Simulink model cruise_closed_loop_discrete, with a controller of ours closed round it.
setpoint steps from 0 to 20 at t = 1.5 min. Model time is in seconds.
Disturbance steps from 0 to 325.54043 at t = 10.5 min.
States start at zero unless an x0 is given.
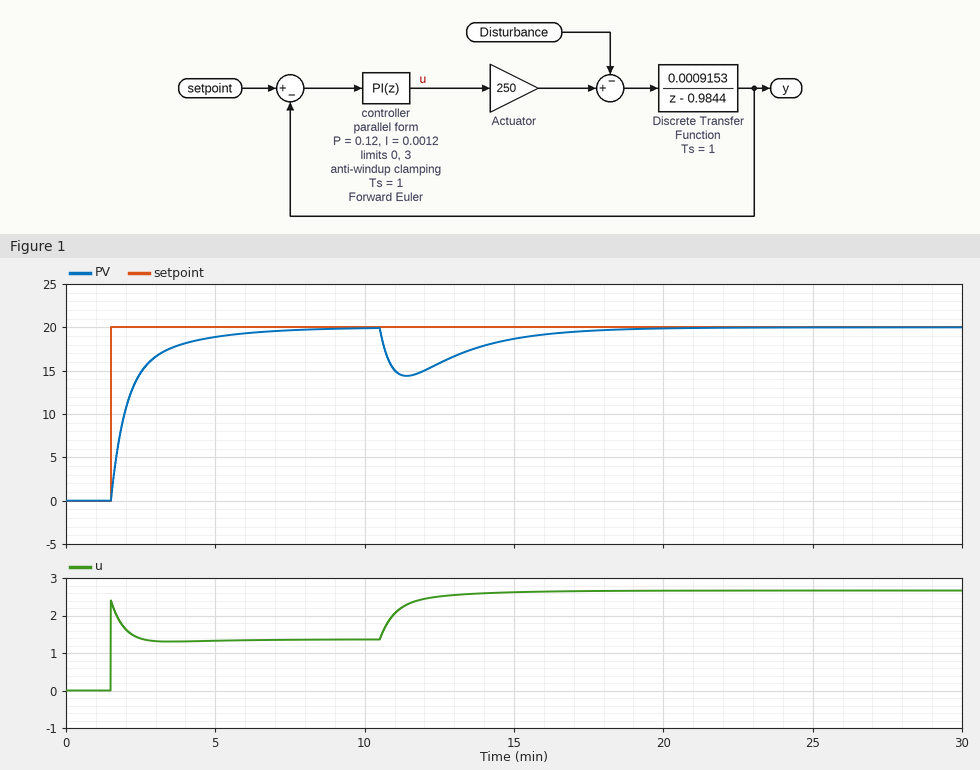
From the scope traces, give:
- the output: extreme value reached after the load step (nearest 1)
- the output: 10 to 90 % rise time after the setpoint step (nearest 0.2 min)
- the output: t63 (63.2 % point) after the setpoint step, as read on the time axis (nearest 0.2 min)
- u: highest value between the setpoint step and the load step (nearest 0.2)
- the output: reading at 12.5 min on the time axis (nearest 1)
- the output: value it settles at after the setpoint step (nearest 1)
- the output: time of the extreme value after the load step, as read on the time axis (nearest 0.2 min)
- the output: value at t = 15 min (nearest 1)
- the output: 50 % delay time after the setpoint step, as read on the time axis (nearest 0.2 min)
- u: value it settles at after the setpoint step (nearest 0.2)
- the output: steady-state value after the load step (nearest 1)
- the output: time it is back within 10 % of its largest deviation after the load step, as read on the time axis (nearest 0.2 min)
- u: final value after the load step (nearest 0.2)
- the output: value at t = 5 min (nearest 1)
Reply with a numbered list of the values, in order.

1. 14
2. 2.2 min
3. 2.2 min
4. 2.4
5. 16
6. 20
7. 11.4 min
8. 19
9. 2.0 min
10. 1.4
11. 20
12. 16.8 min
13. 2.6
14. 19
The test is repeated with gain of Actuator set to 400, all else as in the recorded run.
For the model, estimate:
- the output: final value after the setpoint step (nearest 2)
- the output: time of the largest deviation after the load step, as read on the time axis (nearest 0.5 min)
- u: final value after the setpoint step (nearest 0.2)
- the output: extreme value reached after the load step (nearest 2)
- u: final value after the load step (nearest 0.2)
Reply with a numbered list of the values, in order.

1. 20
2. 11.0 min
3. 0.8
4. 16
5. 1.6
